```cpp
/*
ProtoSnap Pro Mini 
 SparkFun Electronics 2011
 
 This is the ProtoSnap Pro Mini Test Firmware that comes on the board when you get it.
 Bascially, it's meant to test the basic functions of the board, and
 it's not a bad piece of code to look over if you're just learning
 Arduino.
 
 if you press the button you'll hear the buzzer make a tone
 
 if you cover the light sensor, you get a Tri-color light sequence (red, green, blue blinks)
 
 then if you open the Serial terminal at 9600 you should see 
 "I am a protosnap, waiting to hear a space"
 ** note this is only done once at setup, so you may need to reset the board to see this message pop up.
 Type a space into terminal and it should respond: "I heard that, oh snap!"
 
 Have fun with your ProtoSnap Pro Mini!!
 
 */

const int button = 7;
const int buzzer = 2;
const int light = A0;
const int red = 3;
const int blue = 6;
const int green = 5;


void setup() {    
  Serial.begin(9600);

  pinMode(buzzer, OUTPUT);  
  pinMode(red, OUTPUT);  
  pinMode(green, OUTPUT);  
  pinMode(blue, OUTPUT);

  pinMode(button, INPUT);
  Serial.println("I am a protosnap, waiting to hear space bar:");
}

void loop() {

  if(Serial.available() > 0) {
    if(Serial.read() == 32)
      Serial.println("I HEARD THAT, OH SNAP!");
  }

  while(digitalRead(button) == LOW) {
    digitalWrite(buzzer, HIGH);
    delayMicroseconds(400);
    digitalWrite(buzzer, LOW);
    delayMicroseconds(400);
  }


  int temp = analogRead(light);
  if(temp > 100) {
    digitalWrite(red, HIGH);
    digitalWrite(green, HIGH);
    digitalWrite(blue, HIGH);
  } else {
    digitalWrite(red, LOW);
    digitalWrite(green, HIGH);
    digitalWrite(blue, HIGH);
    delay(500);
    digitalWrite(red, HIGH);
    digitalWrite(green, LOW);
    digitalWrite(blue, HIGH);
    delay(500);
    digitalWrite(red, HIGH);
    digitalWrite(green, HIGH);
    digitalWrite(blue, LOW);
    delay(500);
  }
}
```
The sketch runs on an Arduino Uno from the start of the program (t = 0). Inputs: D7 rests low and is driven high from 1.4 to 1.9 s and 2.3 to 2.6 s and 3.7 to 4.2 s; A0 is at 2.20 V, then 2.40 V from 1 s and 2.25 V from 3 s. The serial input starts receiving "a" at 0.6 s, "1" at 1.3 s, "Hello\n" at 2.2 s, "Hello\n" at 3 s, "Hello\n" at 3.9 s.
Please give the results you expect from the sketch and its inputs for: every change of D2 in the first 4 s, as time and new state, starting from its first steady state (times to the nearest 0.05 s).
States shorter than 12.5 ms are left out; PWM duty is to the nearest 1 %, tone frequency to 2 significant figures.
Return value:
0 s tone 1200 Hz; 1.4 s low; 1.9 s tone 1200 Hz; 2.3 s low; 2.6 s tone 1200 Hz; 3.7 s low
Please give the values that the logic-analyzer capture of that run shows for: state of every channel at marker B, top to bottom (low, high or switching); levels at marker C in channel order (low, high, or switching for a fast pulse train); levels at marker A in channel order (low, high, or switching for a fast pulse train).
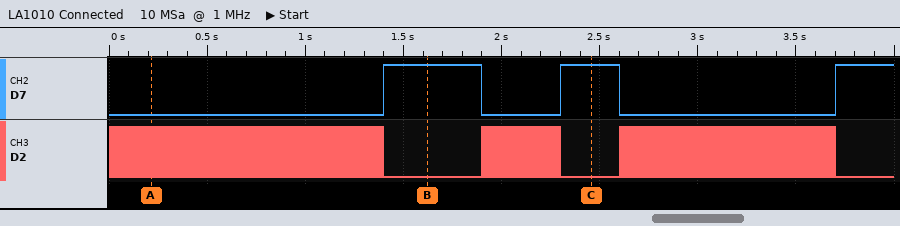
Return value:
D7 high, D2 low
D7 high, D2 low
D7 low, D2 switching
